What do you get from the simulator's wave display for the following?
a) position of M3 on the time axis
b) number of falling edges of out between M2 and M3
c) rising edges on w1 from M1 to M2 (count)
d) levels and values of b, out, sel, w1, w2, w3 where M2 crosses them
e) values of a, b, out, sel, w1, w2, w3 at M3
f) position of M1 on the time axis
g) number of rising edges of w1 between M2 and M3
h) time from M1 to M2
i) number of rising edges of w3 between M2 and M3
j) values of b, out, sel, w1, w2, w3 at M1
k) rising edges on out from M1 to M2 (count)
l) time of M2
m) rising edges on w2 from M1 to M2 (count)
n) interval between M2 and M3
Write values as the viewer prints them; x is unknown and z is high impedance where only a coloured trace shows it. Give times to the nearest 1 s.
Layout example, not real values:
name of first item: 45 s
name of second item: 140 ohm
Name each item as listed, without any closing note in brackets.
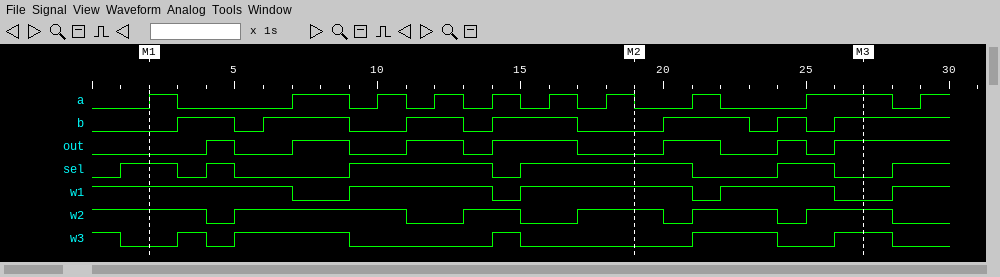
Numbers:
position of M3 on the time axis: 27 s
number of falling edges of out between M2 and M3: 2
rising edges on w1 from M1 to M2: 2
levels and values of b, out, sel, w1, w2, w3 where M2 crosses them: b=0, out=0, sel=1, w1=1, w2=1, w3=0
values of a, b, out, sel, w1, w2, w3 at M3: a=1, b=1, out=1, sel=0, w1=0, w2=1, w3=1
position of M1 on the time axis: 2 s
number of rising edges of w1 between M2 and M3: 1
time from M1 to M2: 17 s
number of rising edges of w3 between M2 and M3: 2
values of b, out, sel, w1, w2, w3 at M1: b=0, out=0, sel=1, w1=1, w2=1, w3=0
rising edges on out from M1 to M2: 4
time of M2: 19 s
rising edges on w2 from M1 to M2: 3
interval between M2 and M3: 8 s
